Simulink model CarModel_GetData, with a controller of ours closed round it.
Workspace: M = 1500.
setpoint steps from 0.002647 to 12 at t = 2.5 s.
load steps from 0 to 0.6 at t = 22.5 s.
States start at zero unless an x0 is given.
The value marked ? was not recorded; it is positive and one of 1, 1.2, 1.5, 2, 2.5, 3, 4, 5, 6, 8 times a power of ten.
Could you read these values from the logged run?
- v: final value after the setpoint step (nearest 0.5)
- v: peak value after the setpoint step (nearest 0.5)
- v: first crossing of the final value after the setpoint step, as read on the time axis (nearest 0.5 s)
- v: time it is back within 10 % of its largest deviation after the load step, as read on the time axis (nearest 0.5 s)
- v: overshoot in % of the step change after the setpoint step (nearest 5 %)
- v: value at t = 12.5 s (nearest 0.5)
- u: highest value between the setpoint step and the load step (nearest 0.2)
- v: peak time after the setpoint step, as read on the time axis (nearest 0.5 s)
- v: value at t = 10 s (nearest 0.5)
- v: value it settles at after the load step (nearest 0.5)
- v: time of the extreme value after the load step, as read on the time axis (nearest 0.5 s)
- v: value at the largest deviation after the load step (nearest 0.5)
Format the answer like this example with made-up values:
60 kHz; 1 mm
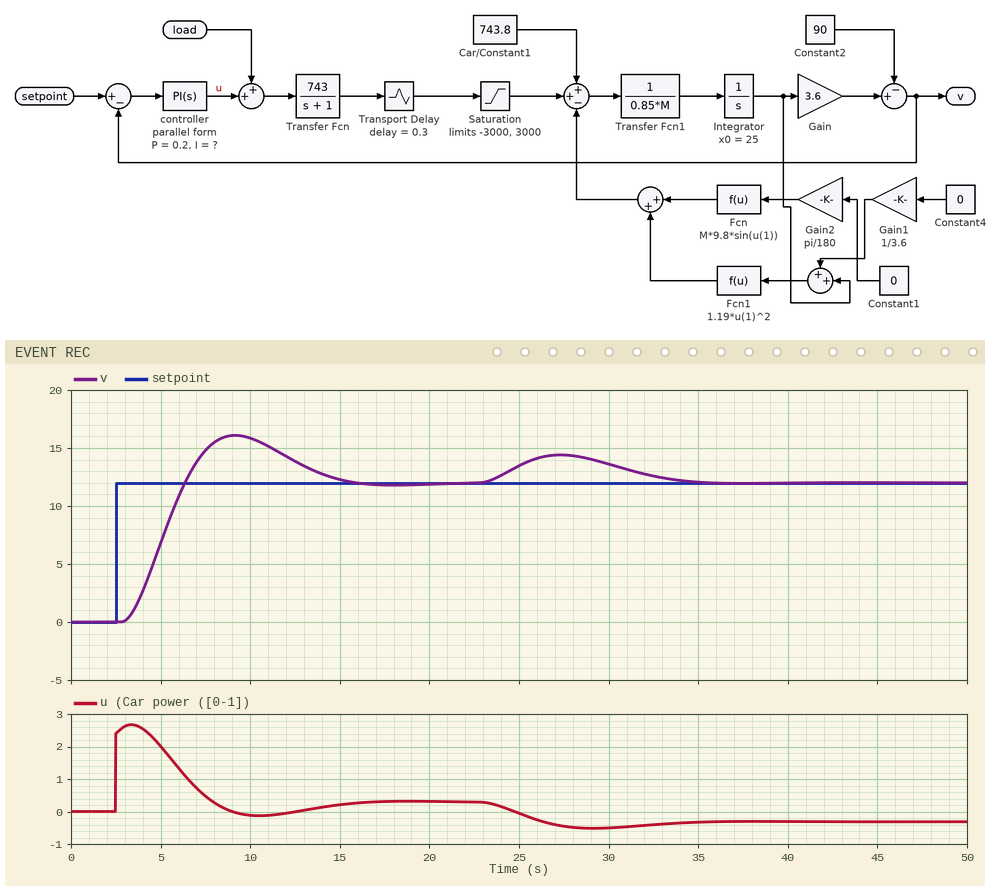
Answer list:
12.0; 16.0; 6.5 s; 34.0 s; 35 %; 14.0; 2.6; 9.0 s; 16.0; 12.0; 27.5 s; 14.5
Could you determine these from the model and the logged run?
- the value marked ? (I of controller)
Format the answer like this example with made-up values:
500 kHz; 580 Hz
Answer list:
0.04
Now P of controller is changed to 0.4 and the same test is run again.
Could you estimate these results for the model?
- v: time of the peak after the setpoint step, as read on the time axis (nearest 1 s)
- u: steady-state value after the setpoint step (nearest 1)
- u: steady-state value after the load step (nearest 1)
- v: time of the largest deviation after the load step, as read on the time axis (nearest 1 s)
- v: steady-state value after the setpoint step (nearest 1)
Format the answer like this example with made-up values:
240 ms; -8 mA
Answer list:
7 s; 0; 0; 26 s; 12
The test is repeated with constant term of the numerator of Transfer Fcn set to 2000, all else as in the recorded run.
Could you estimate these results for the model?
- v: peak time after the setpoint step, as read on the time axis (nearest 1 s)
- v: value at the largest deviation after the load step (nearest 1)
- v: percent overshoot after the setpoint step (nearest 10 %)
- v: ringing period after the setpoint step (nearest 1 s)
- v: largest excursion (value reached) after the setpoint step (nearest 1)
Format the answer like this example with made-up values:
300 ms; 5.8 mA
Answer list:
6 s; 16; 60 %; 7 s; 19
